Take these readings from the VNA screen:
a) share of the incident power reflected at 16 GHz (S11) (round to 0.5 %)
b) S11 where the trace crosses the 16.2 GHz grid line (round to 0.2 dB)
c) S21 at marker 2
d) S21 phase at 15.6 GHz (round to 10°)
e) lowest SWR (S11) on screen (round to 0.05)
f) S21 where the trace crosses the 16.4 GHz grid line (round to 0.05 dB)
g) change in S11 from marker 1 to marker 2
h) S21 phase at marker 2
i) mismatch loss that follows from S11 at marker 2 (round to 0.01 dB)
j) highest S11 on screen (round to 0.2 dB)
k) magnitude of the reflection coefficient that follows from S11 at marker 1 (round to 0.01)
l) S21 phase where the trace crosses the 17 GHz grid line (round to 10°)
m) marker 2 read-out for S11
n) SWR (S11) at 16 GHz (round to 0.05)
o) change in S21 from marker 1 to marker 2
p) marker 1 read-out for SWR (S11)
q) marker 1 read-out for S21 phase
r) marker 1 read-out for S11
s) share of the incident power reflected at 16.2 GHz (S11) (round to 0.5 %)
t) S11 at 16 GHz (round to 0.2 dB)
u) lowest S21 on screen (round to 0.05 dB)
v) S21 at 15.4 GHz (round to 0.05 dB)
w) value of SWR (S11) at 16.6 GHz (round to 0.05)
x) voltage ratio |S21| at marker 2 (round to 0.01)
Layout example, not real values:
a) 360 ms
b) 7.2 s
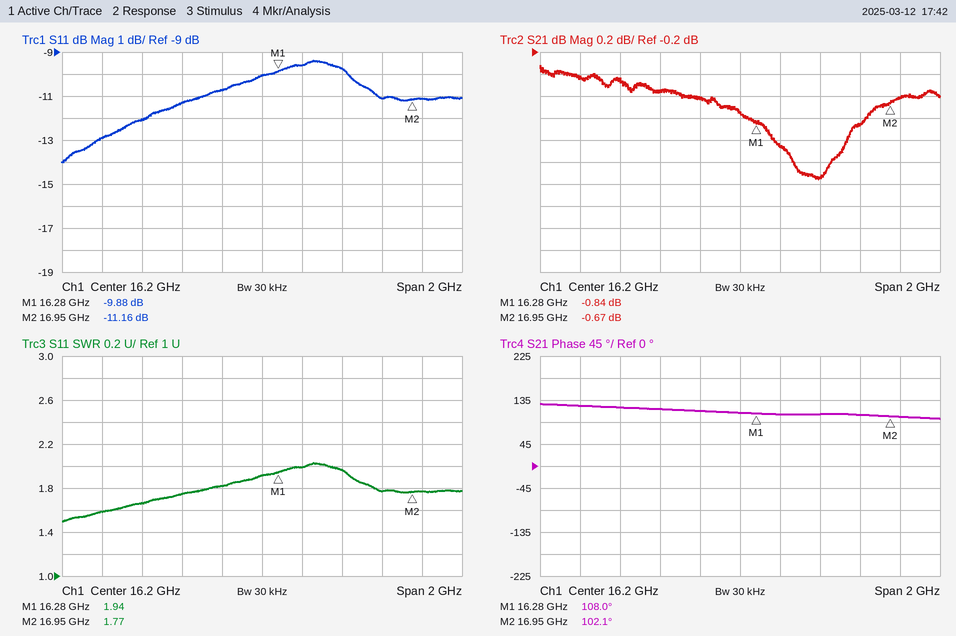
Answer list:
a) 8.5 %
b) -10.0 dB
c) -0.67 dB
d) 120°
e) 1.50
f) -1.05 dB
g) -1.28 dB
h) 102.1°
i) 0.35 dB
j) -9.4 dB
k) 0.32
l) 100°
m) -11.16 dB
n) 1.80
o) 0.17 dB
p) 1.94
q) 108.0°
r) -9.88 dB
s) 10.0 %
t) -10.8 dB
u) -1.35 dB
v) -0.45 dB
w) 1.95
x) 0.93
